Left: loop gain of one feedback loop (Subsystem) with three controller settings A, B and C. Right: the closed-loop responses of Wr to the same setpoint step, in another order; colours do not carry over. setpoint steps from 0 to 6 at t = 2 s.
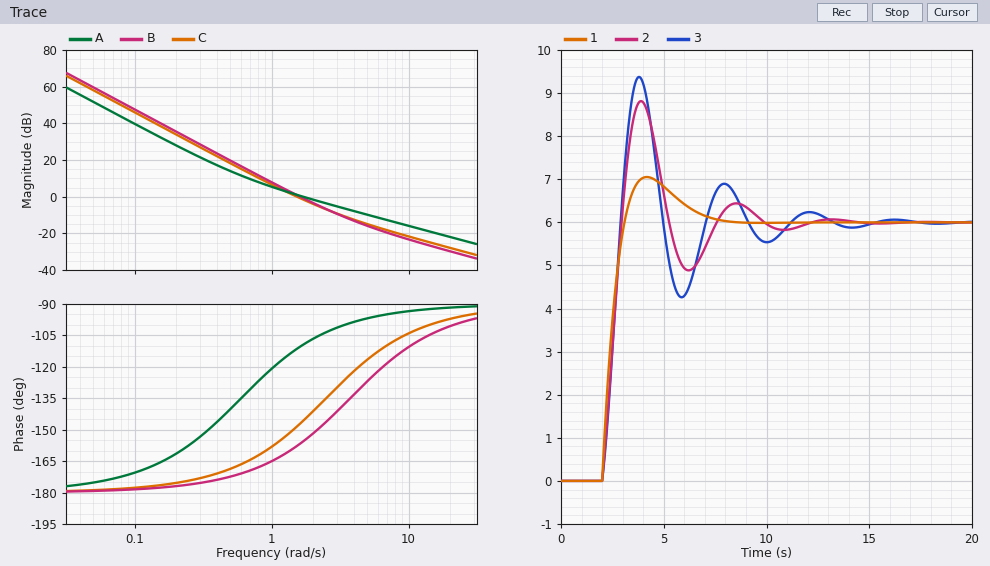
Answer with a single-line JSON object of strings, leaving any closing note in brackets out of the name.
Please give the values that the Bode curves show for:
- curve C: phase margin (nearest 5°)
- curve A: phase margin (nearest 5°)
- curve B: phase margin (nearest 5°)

{"curve C: phase margin": "30°", "curve A: phase margin": "70°", "curve B: phase margin": "25°"}
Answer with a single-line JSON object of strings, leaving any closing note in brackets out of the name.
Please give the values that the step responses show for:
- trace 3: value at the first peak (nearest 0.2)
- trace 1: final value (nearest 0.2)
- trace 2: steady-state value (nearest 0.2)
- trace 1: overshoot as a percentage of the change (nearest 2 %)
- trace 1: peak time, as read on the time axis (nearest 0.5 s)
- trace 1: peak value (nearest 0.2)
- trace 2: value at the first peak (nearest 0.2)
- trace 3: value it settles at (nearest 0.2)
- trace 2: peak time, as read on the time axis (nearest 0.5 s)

{"trace 3: value at the first peak": "9.4", "trace 1: final value": "6.0", "trace 2: steady-state value": "6.0", "trace 1: overshoot as a percentage of the change": "18 %", "trace 1: peak time, as read on the time axis": "4.0 s", "trace 1: peak value": "7.0", "trace 2: value at the first peak": "8.8", "trace 3: value it settles at": "6.0", "trace 2: peak time, as read on the time axis": "4.0 s"}
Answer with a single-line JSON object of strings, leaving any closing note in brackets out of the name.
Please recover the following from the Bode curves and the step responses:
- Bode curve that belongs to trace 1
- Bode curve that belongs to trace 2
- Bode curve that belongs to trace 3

{"Bode curve that belongs to trace 1": "A", "Bode curve that belongs to trace 2": "C", "Bode curve that belongs to trace 3": "B"}
